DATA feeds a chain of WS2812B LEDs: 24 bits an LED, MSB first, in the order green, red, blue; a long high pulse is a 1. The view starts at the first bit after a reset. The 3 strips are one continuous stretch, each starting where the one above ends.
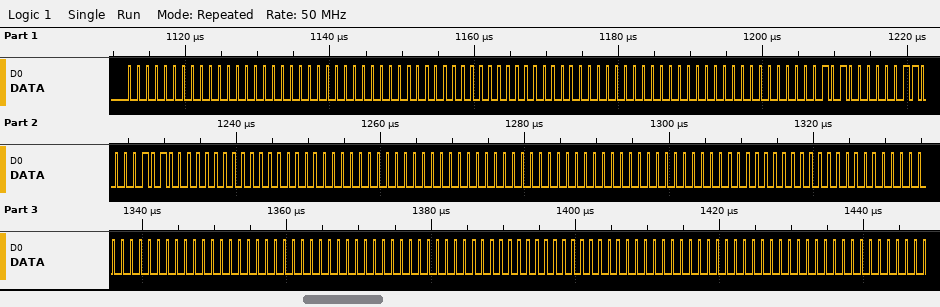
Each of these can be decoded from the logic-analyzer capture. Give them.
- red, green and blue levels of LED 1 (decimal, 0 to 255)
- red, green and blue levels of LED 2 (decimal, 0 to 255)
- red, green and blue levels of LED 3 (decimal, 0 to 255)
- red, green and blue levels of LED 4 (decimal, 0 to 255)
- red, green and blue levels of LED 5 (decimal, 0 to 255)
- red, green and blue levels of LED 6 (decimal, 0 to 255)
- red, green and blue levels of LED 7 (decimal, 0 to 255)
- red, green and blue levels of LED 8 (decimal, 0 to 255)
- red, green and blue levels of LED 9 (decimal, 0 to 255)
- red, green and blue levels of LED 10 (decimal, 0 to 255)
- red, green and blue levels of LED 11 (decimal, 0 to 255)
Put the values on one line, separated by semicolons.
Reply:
0, 0, 0; 0, 0, 0; 0, 0, 0; 3, 5, 10; 0, 0, 0; 0, 0, 0; 0, 0, 0; 0, 0, 0; 0, 0, 0; 0, 0, 0; 0, 0, 0
